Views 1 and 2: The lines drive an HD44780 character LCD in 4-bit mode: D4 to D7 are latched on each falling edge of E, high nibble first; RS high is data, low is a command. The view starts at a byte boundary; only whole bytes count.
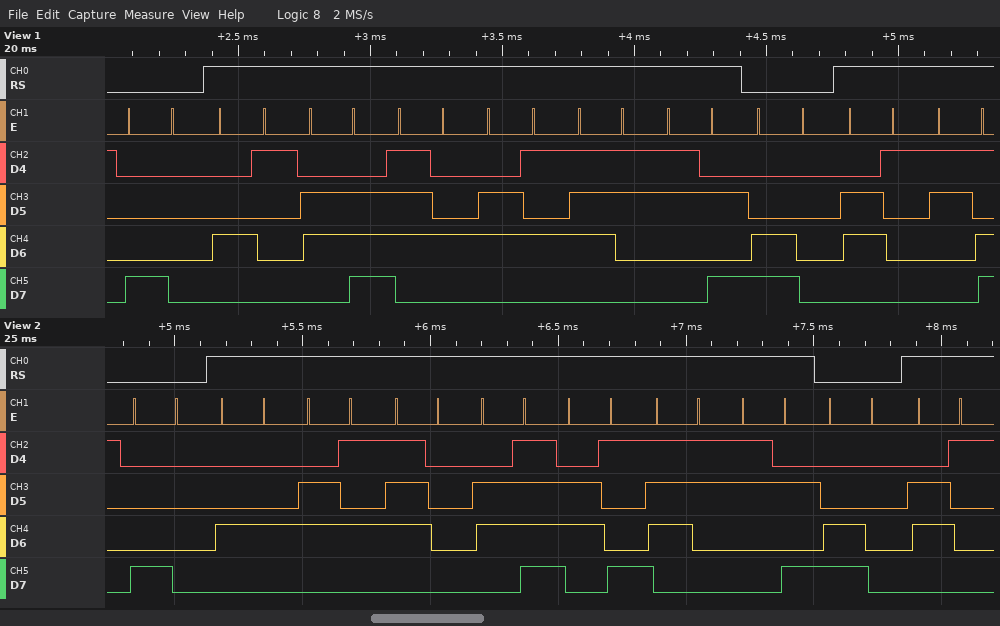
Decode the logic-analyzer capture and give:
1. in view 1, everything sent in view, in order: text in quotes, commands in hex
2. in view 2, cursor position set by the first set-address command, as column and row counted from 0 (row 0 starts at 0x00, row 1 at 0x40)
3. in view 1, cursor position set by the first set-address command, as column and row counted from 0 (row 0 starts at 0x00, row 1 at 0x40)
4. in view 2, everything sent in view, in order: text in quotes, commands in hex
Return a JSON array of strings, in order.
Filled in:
["0x80 \"Antes:\" 0xC0 \"a=\"", "column 0, row 0", "column 0, row 0", "0x80 \"Depois:\" 0xC0 \"a\""]
